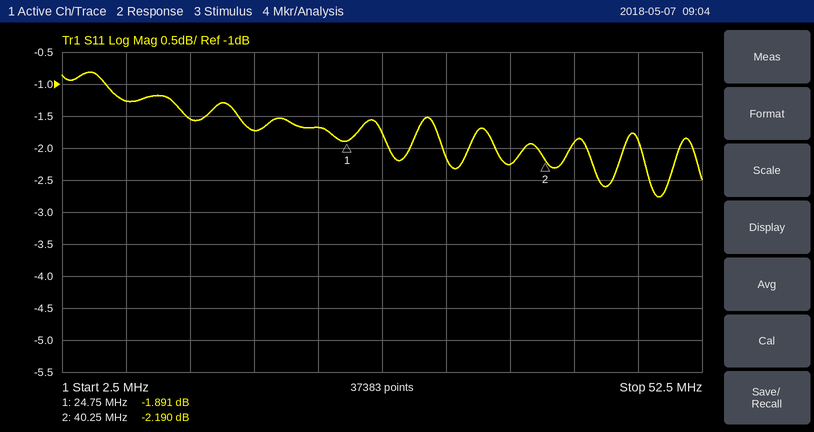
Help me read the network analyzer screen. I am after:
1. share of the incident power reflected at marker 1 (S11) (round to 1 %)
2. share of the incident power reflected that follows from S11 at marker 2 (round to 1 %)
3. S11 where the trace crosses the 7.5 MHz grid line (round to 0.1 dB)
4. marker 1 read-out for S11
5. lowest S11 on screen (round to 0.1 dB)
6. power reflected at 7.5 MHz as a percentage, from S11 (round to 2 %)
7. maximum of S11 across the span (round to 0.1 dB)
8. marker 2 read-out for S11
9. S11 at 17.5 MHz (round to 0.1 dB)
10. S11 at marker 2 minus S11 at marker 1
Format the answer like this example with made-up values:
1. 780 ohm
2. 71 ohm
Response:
1. 65 %
2. 60 %
3. -1.3 dB
4. -1.891 dB
5. -2.8 dB
6. 74 %
7. -0.8 dB
8. -2.190 dB
9. -1.7 dB
10. -0.299 dB
